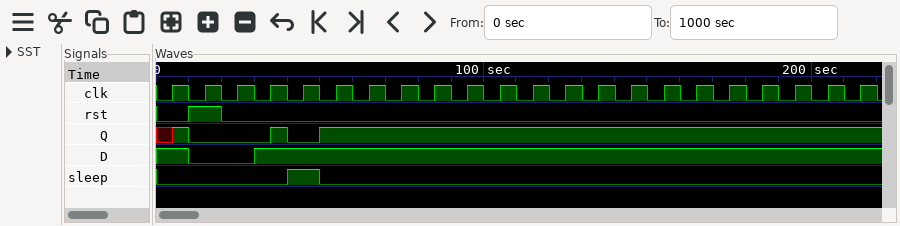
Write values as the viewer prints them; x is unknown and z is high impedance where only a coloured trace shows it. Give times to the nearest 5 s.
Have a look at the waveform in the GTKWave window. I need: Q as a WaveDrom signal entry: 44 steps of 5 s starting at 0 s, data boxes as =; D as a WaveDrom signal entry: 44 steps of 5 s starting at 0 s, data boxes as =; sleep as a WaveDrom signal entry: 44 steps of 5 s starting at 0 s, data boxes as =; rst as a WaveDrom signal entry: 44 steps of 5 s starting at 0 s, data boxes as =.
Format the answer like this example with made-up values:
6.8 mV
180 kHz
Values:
{name: 'Q', wave: 'x10....10.1.................................'}
{name: 'D', wave: '1.0...1.....................................'}
{name: 'sleep', wave: '0.......1.0.................................'}
{name: 'rst', wave: '0.1.0.......................................'}
